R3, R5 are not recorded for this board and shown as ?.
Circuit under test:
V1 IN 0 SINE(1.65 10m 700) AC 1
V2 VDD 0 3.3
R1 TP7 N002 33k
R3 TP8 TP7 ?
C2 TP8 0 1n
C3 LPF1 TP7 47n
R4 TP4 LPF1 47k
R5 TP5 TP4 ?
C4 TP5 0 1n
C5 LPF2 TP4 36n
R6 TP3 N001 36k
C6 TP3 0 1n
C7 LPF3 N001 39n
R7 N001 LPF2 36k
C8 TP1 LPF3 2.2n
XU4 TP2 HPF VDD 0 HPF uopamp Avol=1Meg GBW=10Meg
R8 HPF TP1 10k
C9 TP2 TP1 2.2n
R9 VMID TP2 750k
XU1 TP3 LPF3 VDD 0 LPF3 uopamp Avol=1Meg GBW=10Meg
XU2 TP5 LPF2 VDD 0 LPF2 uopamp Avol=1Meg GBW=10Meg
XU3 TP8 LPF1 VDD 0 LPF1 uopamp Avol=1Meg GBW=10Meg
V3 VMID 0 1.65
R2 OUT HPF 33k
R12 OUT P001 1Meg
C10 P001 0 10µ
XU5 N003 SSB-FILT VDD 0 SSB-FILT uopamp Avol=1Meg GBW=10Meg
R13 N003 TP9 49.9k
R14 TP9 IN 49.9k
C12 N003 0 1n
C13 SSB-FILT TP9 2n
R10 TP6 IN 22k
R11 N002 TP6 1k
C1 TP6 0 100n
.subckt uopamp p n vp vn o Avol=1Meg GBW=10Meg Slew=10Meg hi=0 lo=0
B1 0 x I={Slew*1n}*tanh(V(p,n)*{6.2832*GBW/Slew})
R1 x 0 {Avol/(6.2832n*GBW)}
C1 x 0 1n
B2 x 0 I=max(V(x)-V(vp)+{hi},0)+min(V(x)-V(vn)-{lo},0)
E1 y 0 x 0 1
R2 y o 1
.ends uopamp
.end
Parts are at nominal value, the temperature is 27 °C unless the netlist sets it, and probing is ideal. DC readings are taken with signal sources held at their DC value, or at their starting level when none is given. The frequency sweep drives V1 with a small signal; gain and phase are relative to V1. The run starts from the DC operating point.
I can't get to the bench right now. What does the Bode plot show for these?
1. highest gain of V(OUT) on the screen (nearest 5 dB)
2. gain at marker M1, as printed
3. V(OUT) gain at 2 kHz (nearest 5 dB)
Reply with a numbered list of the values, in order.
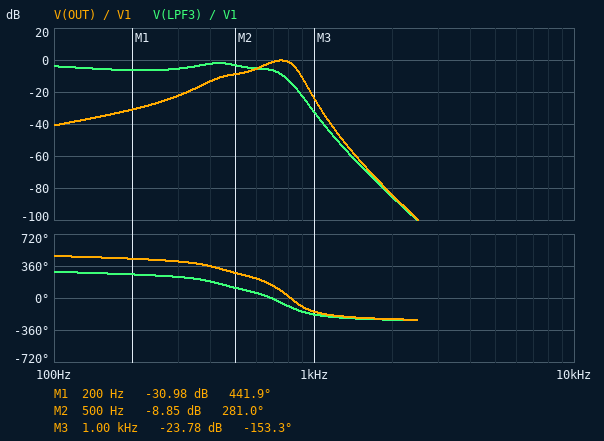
1. 0 dB
2. -30.98 dB
3. -85 dB
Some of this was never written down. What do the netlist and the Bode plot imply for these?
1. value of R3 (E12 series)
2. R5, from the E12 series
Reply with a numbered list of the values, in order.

1. 82 kΩ
2. 22 kΩ
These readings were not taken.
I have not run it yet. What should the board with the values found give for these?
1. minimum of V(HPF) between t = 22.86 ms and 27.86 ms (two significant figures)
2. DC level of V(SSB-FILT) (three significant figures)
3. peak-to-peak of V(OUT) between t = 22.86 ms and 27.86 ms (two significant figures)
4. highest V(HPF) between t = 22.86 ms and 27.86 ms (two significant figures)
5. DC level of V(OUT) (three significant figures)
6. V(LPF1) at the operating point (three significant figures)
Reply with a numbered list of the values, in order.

1. 1.6 V
2. 1.65 V
3. 18 mV
4. 1.7 V
5. 1.65 V
6. 1.65 V
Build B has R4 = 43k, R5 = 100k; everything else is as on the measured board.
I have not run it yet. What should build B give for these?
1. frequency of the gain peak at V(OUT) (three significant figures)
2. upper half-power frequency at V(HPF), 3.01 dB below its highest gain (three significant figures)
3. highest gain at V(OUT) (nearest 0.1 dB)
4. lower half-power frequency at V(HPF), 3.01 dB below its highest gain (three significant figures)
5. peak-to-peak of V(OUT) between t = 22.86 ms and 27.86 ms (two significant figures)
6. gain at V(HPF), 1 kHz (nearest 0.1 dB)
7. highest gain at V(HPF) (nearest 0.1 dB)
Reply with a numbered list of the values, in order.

1. 424 Hz
2. 495 Hz
3. -5.8 dB
4. 371 Hz
5. 3.5 mV
6. -41.7 dB
7. -5.6 dB
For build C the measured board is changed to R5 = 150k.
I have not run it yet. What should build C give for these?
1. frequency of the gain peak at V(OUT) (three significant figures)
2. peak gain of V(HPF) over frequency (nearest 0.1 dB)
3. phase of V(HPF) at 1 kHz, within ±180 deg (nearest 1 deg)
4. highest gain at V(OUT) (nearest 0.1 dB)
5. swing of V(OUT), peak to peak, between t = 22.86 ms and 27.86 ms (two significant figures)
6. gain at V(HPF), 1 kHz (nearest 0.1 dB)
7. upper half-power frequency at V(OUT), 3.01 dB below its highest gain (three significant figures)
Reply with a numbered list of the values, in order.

1. 366 Hz
2. -12.7 dB
3. 172 deg
4. -13.0 dB
5. 1.8 mV
6. -46.6 dB
7. 488 Hz
